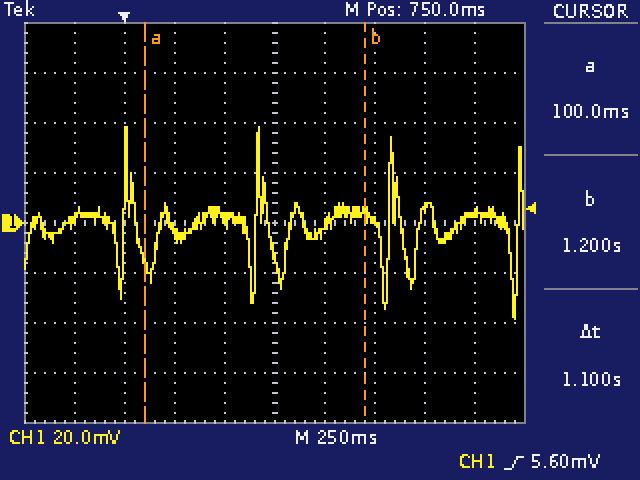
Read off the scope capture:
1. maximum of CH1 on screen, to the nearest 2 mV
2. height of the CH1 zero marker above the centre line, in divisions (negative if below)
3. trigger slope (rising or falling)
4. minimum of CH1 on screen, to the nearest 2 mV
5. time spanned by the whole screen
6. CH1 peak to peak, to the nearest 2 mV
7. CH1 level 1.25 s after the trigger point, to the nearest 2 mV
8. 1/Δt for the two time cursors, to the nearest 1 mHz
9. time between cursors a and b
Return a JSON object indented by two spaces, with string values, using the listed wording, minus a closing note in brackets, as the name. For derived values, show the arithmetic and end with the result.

{
  "maximum of CH1 on screen, to the nearest 2 mV": "38 mV",
  "height of the CH1 zero marker above the centre line, in divisions": "0.0 div",
  "trigger slope": "rising",
  "minimum of CH1 on screen, to the nearest 2 mV": "-38 mV",
  "time spanned by the whole screen": "2.5 s",
  "CH1 peak to peak, to the nearest 2 mV": "38 mV − (-38 mV) = 76 mV",
  "CH1 level 1.25 s after the trigger point, to the nearest 2 mV": "0 mV",
  "1/Δt for the two time cursors, to the nearest 1 mHz": "1 / 1.1 s ≈ 909 mHz",
  "time between cursors a and b": "1.1 s"
}
